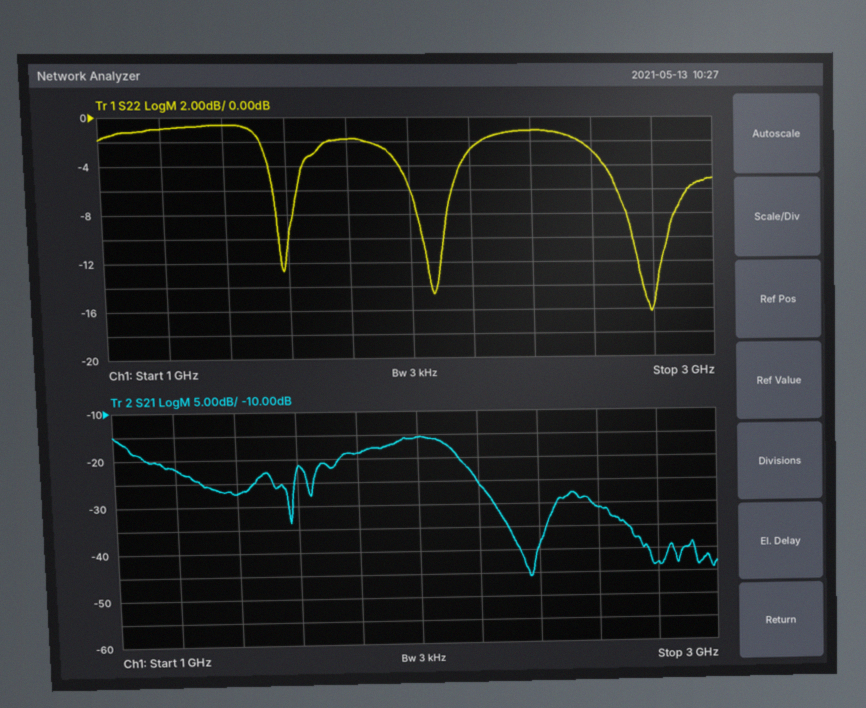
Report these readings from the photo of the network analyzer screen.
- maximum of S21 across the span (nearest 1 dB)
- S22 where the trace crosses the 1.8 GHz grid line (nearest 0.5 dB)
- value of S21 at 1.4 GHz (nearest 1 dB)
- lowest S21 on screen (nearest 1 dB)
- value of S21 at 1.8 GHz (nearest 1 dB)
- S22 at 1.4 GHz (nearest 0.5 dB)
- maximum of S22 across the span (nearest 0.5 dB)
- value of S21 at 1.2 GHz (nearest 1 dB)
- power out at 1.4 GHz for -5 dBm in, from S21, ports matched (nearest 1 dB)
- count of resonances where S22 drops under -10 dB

-15 dB
-2.0 dB
-27 dB
-46 dB
-19 dB
-0.5 dB
-0.5 dB
-22 dB
-32 dBm
3
